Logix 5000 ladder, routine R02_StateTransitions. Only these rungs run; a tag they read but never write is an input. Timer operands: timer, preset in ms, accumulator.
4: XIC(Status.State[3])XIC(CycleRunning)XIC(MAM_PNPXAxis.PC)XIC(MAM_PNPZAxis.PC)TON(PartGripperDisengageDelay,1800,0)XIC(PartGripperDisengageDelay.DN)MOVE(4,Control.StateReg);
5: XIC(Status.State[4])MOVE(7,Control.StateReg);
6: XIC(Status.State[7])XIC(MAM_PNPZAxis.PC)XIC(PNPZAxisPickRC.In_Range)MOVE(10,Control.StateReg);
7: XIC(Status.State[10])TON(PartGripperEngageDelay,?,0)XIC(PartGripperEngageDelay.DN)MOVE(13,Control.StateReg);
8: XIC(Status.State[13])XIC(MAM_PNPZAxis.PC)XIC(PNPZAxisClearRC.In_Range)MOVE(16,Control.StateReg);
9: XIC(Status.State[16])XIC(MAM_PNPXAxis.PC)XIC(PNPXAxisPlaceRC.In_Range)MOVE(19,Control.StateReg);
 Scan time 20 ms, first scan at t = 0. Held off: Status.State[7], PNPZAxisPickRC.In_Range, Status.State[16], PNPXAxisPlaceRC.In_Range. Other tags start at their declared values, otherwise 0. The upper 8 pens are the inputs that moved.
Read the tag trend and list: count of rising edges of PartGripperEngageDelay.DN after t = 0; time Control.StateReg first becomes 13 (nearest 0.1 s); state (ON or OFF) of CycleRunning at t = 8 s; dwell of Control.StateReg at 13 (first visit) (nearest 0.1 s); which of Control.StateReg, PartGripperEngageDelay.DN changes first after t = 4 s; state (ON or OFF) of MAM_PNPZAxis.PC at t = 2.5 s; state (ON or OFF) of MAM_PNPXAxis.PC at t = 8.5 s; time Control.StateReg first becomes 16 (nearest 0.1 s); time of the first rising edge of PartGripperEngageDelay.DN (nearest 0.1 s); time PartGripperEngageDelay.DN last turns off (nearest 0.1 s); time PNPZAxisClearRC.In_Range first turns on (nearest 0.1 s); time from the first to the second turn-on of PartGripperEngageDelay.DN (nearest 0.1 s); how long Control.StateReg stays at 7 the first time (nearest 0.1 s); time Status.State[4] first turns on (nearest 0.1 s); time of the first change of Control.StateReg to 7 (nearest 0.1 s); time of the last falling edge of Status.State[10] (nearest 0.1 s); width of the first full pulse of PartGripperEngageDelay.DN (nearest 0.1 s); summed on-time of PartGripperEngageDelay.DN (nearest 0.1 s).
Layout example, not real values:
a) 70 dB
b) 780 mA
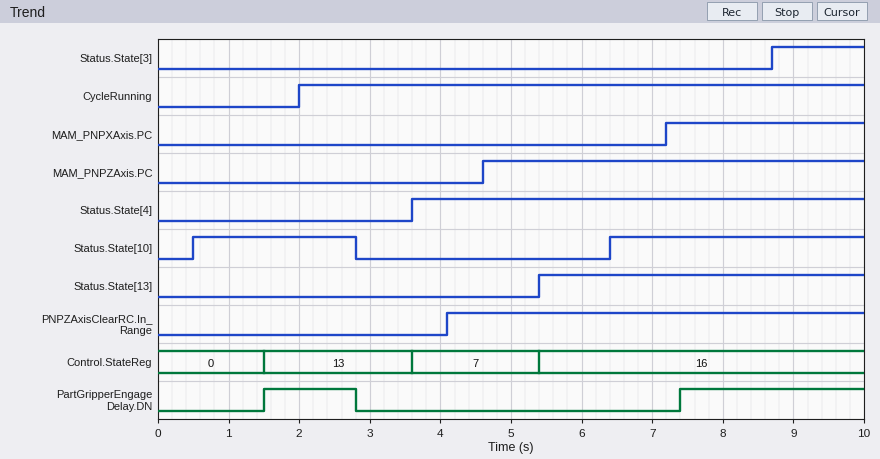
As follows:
a) 2
b) 1.5 s
c) ON
d) 2.1 s
e) Control.StateReg
f) OFF
g) ON
h) 5.4 s
i) 1.5 s
j) 2.8 s
k) 4.1 s
l) 5.9 s
m) 1.8 s
n) 3.6 s
o) 3.6 s
p) 2.8 s
q) 1.3 s
r) 3.9 s
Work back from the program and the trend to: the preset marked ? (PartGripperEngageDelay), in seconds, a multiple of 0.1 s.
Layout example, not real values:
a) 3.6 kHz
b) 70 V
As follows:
a) 1.0 s
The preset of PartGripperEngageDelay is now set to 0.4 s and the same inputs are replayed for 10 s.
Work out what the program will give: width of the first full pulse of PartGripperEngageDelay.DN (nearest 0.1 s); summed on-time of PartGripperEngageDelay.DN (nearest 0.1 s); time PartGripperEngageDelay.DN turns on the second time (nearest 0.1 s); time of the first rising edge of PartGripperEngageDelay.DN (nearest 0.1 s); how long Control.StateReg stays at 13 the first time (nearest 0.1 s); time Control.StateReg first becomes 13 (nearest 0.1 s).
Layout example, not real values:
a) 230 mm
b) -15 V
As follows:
a) 1.9 s
b) 5.1 s
c) 6.8 s
d) 0.9 s
e) 2.7 s
f) 0.9 s
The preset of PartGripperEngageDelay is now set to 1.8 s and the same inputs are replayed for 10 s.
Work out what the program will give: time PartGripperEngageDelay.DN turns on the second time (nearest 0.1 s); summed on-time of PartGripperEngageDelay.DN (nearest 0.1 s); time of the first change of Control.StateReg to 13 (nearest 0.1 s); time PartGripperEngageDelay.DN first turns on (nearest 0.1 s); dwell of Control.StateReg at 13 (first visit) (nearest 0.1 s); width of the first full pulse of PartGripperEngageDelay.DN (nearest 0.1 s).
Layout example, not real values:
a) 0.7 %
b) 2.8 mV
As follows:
a) 8.2 s
b) 2.3 s
c) 2.3 s
d) 2.3 s
e) 1.3 s
f) 0.5 s
